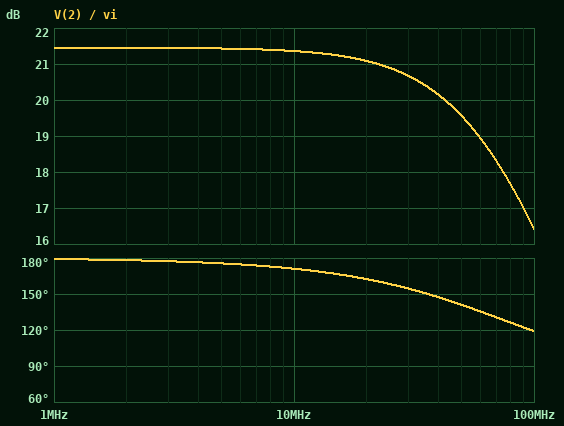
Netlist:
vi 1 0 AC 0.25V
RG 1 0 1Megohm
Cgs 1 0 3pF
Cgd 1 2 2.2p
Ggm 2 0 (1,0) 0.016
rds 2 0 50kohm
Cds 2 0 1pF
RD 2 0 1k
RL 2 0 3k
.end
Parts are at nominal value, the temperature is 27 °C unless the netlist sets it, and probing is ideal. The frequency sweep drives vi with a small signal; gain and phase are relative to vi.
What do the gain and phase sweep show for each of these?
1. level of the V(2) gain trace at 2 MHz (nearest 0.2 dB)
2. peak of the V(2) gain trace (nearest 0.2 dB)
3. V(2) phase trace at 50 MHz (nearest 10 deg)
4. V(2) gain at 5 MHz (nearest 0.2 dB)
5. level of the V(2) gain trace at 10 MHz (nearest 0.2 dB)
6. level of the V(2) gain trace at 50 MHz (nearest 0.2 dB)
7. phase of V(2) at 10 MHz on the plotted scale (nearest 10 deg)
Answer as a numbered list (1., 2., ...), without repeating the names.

1. 21.4 dB
2. 21.4 dB
3. 140 deg
4. 21.4 dB
5. 21.4 dB
6. 19.6 dB
7. 170 deg
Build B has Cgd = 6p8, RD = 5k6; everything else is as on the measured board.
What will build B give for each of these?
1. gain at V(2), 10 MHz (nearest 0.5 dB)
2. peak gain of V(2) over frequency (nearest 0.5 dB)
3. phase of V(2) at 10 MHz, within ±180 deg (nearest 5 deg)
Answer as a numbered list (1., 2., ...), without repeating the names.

1. 27.0 dB
2. 29.5 dB
3. 135 deg
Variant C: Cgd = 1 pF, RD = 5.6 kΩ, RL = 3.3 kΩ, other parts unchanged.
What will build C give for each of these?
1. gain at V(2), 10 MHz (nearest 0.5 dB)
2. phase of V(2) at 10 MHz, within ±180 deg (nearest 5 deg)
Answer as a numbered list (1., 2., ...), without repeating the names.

1. 30.0 dB
2. 165 deg
